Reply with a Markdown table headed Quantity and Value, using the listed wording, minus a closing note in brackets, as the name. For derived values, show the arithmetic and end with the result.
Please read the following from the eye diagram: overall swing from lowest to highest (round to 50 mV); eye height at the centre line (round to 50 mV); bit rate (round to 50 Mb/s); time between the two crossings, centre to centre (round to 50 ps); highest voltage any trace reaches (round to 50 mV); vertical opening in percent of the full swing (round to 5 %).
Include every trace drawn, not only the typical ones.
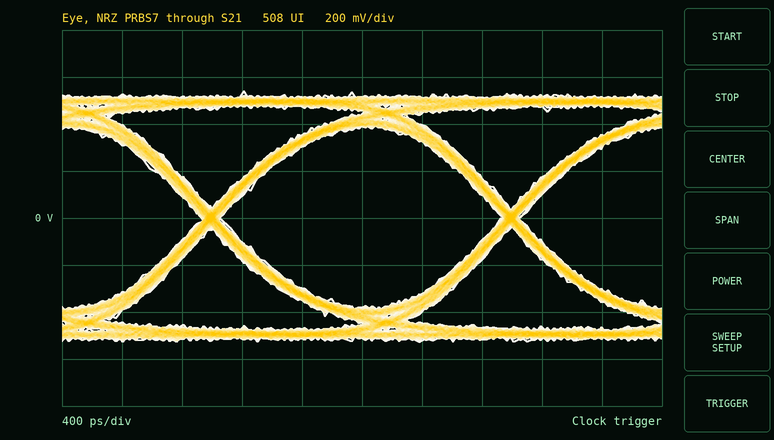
| Quantity | Value |
|---|---|
| overall swing from lowest to highest | 1.05 V |
| eye height at the centre line | 750 mV |
| bit rate | 500 Mb/s |
| time between the two crossings, centre to centre | 2.00 ns |
| highest voltage any trace reaches | 550 mV |
| vertical opening in percent of the full swing | 750 mV / 1.05 V ≈ 71.4 %, so 70 % to the nearest 5 % |
